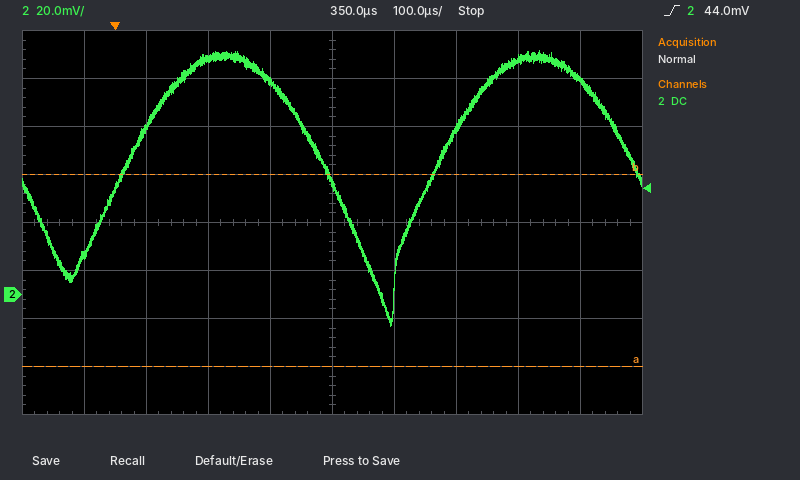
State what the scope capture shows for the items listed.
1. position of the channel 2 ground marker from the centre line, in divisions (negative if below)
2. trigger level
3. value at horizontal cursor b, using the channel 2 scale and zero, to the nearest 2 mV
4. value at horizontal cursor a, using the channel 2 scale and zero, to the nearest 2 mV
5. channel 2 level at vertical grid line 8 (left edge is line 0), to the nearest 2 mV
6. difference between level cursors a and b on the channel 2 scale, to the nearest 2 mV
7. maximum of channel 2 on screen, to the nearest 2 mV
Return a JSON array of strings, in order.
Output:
["-1.5 div", "44.0 mV", "50 mV", "-30 mV", "98 mV", "80 mV", "102 mV"]
